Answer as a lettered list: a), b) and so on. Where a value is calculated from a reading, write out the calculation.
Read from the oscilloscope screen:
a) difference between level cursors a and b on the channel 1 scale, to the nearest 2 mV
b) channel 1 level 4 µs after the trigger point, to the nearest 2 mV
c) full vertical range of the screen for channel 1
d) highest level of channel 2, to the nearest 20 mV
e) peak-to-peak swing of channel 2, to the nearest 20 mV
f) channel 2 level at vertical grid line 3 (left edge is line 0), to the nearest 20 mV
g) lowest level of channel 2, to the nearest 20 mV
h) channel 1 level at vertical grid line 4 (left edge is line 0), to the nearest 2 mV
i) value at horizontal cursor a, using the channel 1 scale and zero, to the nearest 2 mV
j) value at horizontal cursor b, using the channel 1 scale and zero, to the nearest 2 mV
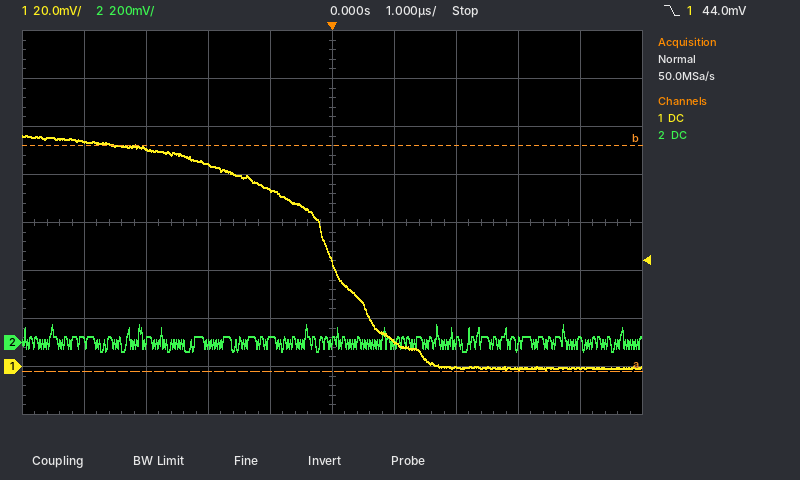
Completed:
a) 94 mV
b) 0 mV
c) 160 mV
d) 80 mV
e) 80 mV − (-40 mV) = 120 mV
f) 0 mV
g) -40 mV
h) 74 mV
i) -2 mV
j) 92 mV
